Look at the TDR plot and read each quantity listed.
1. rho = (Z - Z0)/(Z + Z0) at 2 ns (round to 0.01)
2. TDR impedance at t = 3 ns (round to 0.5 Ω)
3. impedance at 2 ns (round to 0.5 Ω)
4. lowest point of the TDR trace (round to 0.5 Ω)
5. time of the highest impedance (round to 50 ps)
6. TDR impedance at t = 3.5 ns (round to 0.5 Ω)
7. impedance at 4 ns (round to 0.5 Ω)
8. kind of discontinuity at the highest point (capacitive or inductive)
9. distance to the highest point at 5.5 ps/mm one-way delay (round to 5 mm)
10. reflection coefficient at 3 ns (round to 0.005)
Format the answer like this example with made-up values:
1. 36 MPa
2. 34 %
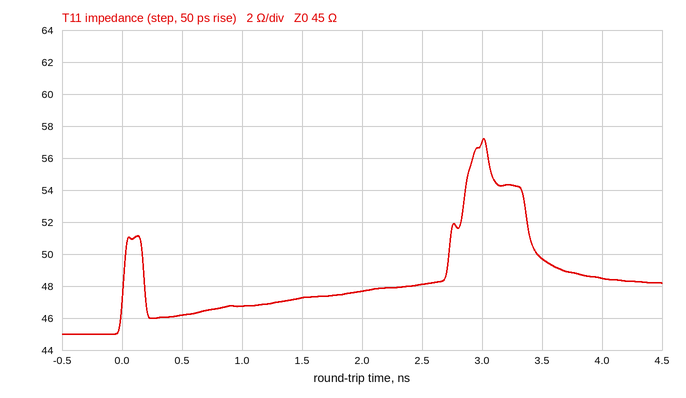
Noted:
1. +0.03
2. 57.0 Ω
3. 47.5 Ω
4. 45.0 Ω
5. 3.00 ns
6. 49.5 Ω
7. 48.5 Ω
8. inductive
9. 275 mm
10. +0.120
